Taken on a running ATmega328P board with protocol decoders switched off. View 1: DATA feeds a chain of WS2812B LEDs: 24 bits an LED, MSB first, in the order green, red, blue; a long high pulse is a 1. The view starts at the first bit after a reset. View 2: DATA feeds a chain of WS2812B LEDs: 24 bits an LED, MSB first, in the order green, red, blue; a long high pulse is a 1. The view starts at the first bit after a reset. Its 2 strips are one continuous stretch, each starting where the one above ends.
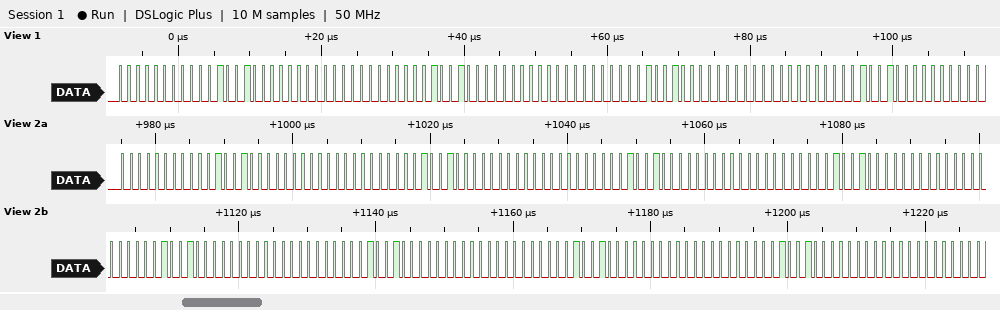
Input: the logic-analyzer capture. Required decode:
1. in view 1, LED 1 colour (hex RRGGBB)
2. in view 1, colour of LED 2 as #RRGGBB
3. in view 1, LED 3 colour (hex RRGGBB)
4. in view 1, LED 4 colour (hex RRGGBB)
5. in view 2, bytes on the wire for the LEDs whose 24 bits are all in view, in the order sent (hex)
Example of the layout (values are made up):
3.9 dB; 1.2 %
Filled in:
#120000; #120000; #120000; #120000; 00 12 00 00 12 00 00 12 00 00 12 00 00 12 00 00 12 00 00 12 00 00 12 00
